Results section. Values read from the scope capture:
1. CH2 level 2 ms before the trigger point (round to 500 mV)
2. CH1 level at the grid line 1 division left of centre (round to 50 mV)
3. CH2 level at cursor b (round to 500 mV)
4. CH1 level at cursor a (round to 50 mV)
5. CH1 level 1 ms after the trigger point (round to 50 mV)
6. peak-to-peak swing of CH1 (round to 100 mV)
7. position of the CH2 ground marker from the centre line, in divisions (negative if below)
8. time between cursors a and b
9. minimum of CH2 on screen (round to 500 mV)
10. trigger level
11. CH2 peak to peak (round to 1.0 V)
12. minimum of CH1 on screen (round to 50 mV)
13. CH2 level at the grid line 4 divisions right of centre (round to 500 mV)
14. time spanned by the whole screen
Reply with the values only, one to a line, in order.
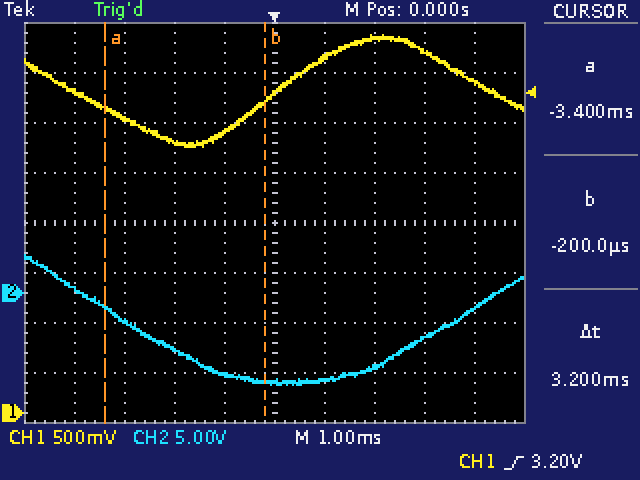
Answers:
-5.5 V
2.80 V
-9.0 V
3.05 V
3.55 V
1.10 V
-1.4 div
3.2 ms
-9.0 V
3.20 V
13.0 V
2.65 V
-1.5 V
10 ms
